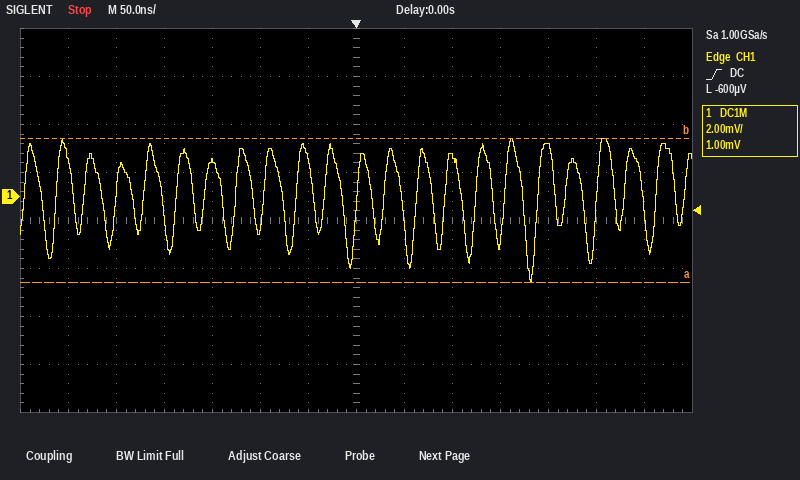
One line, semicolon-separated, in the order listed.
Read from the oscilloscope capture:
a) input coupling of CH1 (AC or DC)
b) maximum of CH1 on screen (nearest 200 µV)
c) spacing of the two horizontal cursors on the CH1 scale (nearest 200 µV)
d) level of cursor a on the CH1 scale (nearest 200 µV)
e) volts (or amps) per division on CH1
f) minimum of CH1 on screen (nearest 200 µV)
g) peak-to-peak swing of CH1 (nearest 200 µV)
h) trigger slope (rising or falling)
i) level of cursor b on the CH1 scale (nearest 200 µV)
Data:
DC; 2.4 mV; 6.0 mV; -3.6 mV; 2 mV; -3.6 mV; 6.0 mV; rising; 2.4 mV
